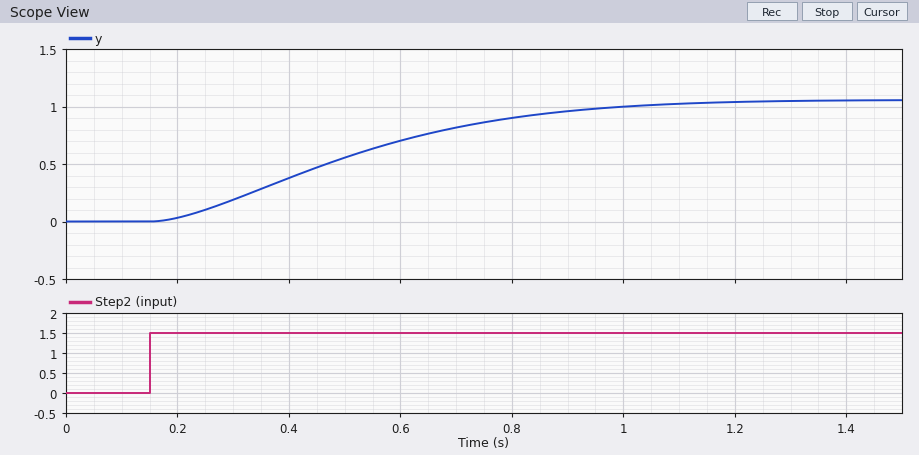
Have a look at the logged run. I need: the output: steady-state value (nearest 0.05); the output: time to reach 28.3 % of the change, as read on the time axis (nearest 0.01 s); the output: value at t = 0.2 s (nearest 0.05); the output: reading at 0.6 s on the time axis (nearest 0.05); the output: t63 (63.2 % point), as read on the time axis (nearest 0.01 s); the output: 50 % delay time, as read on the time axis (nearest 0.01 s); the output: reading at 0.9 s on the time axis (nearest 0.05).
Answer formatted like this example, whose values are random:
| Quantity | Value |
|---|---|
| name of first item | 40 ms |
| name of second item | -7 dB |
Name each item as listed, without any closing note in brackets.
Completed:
| Quantity | Value |
|---|---|
| the output: steady-state value | 1.05 |
| the output: time to reach 28.3 % of the change, as read on the time axis | 0.36 s |
| the output: value at t = 0.2 s | 0.05 |
| the output: reading at 0.6 s on the time axis | 0.70 |
| the output: t63 (63.2 % point), as read on the time axis | 0.57 s |
| the output: 50 % delay time, as read on the time axis | 0.48 s |
| the output: reading at 0.9 s on the time axis | 0.95 |
